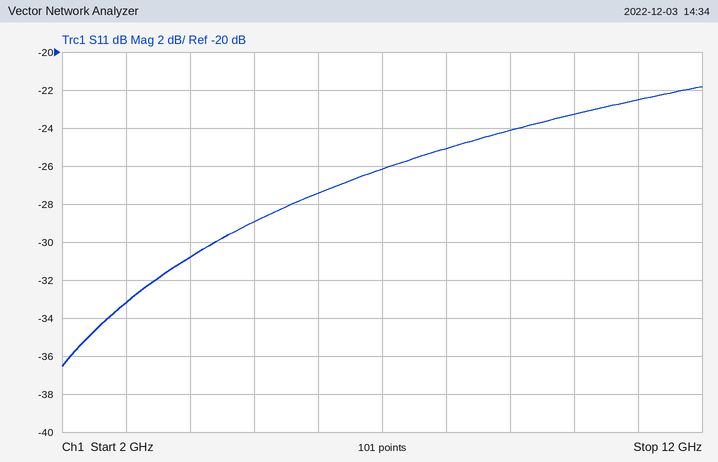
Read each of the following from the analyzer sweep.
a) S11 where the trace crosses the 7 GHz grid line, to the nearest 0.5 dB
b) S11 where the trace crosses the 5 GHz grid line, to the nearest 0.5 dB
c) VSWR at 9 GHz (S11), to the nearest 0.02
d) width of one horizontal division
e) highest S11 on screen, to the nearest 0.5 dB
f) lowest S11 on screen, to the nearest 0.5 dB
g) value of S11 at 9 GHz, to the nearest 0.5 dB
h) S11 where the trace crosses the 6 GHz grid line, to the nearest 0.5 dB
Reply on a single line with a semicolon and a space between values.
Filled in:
-26.0 dB; -29.0 dB; 1.14; 1 GHz; -22.0 dB; -36.5 dB; -24.0 dB; -27.5 dB
